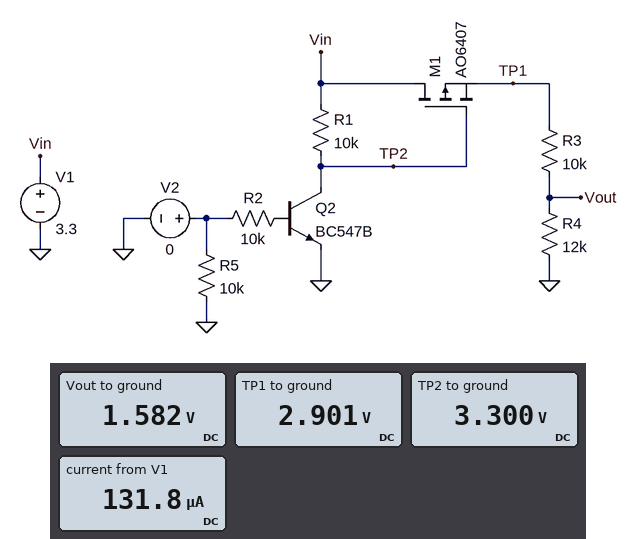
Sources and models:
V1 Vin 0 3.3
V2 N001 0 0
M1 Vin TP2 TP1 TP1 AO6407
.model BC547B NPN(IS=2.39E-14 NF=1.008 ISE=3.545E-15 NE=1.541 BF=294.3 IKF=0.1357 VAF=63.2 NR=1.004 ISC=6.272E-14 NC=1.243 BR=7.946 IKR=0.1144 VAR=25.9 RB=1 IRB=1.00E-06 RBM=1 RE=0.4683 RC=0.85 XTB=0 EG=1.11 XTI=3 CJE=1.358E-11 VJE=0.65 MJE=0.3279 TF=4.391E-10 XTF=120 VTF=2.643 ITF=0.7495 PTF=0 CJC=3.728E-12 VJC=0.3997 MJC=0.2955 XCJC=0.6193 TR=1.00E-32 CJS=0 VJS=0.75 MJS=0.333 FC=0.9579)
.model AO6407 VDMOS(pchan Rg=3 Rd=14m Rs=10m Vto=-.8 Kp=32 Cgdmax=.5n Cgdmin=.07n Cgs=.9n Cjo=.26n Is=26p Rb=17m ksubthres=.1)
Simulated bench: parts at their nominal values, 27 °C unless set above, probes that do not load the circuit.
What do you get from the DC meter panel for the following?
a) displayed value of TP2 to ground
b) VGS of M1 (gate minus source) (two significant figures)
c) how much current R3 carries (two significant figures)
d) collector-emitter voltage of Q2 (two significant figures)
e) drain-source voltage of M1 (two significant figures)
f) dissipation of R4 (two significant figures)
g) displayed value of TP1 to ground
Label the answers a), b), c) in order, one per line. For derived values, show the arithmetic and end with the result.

a) 3.300 V
b) 3.3 V - 2.901 V = 400 mV
c) (2.901 V - 1.582 V) / 10 kΩ = 130 µA
d) 3.3 V = 3.3 V
e) 3.3 V - 2.901 V = 400 mV
f) (1.582 V)^2 / 12 kΩ = 210 µW
g) 2.901 V
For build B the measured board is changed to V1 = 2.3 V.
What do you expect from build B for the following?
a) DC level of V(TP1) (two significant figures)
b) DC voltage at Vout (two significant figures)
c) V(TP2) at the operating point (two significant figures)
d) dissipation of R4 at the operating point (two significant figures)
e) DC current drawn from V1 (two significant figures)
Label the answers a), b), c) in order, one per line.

a) 1.9 V
b) 1.0 V
c) 2.3 V
d) 91 µW
e) 87 µA
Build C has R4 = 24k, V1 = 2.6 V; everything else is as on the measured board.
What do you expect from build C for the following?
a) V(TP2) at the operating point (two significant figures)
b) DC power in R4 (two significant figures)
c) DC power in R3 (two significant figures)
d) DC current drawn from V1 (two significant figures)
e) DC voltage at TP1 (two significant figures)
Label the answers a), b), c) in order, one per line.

a) 2.6 V
b) 100 µW
c) 43 µW
d) 65 µA
e) 2.2 V
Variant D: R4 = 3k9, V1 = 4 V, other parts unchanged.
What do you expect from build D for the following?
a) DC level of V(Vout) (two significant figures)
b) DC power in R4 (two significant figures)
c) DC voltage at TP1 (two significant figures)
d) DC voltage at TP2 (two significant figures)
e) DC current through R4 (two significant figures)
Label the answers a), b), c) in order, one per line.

a) 1.0 V
b) 260 µW
c) 3.6 V
d) 4.0 V
e) 260 µA
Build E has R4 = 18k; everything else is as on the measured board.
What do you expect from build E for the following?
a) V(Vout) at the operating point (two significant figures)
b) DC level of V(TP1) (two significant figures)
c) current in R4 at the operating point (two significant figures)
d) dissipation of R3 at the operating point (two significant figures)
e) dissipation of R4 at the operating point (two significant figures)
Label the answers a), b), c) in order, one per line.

a) 1.9 V
b) 2.9 V
c) 100 µA
d) 110 µW
e) 190 µW
